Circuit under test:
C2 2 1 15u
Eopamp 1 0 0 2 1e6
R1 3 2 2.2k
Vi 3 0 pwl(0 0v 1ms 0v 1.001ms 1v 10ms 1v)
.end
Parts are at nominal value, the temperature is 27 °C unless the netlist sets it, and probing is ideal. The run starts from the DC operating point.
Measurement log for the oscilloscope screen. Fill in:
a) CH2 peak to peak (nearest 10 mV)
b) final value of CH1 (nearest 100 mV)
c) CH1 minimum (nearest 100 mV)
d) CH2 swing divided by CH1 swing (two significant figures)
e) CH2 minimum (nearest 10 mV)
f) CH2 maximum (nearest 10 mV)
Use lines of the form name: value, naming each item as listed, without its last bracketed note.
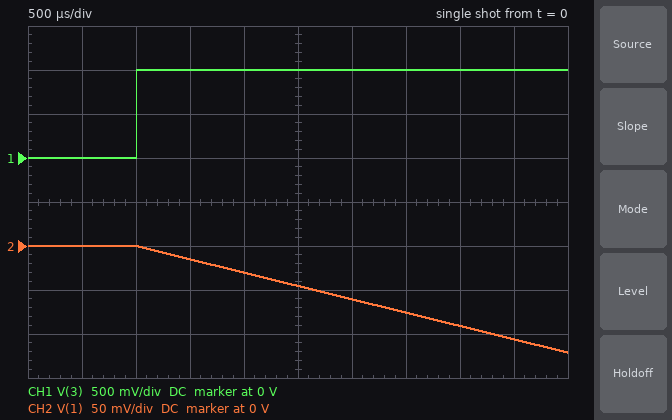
CH2 peak to peak: 120 mV
final value of CH1: 1.0 V
CH1 minimum: 0 V
CH2 swing divided by CH1 swing: 0.12
CH2 minimum: -120 mV
CH2 maximum: 0 V
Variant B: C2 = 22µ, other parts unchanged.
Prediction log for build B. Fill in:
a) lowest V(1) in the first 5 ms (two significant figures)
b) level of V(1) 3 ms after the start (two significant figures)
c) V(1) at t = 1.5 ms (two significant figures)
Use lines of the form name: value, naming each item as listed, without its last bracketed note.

lowest V(1) in the first 5 ms: -83 mV
level of V(1) 3 ms after the start: -41 mV
V(1) at t = 1.5 ms: -10 mV
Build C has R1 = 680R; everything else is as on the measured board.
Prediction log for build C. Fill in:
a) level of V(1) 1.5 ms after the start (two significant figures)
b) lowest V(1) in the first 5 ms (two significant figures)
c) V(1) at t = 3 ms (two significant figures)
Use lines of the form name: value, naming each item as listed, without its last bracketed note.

level of V(1) 1.5 ms after the start: -49 mV
lowest V(1) in the first 5 ms: -390 mV
V(1) at t = 3 ms: -200 mV
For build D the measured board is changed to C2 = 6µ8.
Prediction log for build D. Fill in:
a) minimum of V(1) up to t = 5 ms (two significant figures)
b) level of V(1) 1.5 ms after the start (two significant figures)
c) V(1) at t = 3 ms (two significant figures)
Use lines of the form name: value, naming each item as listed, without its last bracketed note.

minimum of V(1) up to t = 5 ms: -270 mV
level of V(1) 1.5 ms after the start: -33 mV
V(1) at t = 3 ms: -130 mV
